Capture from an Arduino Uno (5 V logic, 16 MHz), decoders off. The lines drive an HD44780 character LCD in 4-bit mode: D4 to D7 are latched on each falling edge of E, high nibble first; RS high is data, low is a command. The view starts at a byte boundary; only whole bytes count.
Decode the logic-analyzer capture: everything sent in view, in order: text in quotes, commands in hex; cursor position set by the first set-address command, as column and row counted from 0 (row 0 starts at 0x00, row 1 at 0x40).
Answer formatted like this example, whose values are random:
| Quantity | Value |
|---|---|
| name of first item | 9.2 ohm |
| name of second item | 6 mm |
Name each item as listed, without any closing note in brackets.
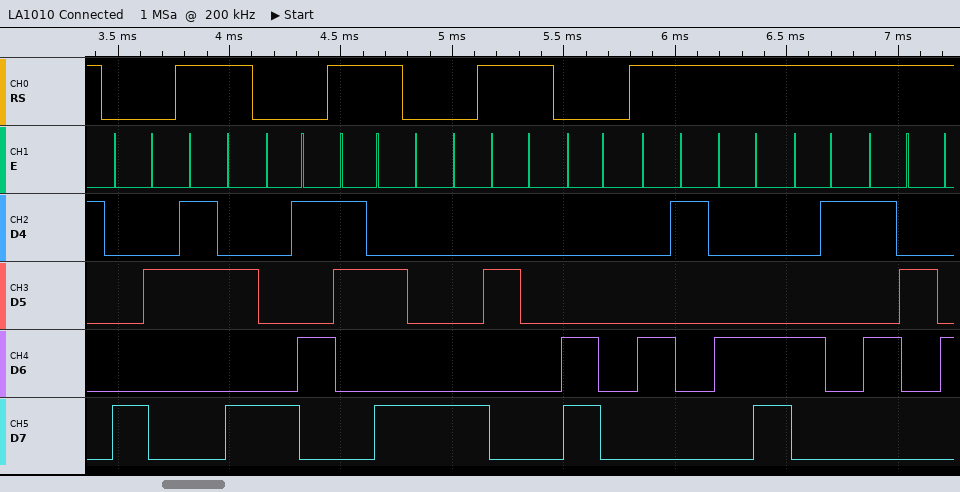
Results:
| Quantity | Value |
|---|---|
| everything sent in view, in order: text in quotes, commands in hex | 0x82 ":" 0x85 ":" 0x88 " " 0xC0 "ALAR" |
| cursor position set by the first set-address command, as column and row counted from 0 | column 2, row 0 |
